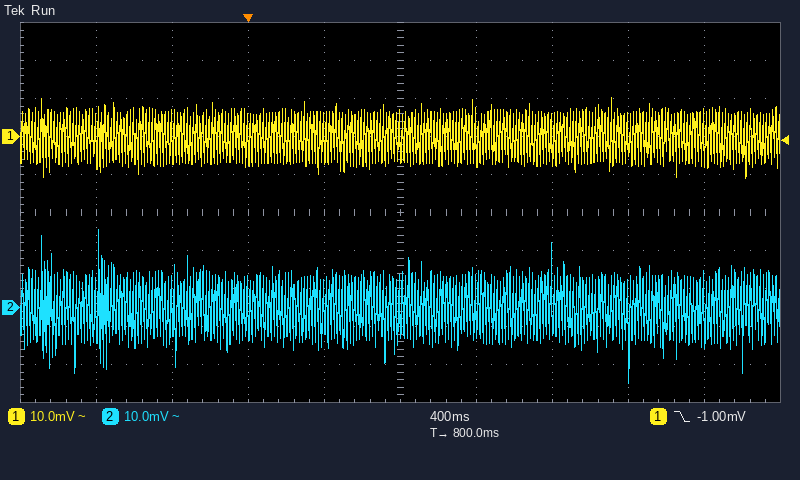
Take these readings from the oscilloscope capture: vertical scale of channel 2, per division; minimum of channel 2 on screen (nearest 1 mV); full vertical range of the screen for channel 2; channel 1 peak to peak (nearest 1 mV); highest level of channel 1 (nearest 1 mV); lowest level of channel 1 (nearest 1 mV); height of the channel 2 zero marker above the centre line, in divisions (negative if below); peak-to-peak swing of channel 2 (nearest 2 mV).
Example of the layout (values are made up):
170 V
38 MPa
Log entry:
10 mV
-20 mV
100 mV
21 mV
10 mV
-11 mV
-2.5 div
40 mV
